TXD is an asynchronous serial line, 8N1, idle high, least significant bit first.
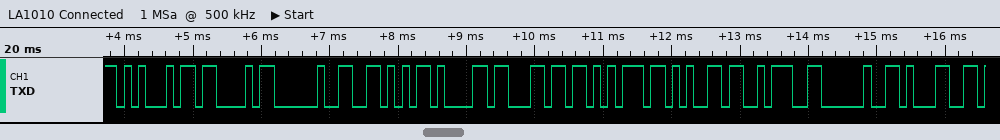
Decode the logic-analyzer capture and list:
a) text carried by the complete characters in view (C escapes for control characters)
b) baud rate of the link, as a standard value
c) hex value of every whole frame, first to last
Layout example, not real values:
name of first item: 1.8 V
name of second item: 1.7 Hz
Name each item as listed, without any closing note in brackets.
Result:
text carried by the complete characters in view: "EC Value: 1"
baud rate of the link, as a standard value: 9600 baud
hex value of every whole frame, first to last: 0x45 0x43 0x20 0x56 0x61 0x6C 0x75 0x65 0x3A 0x20 0x31
